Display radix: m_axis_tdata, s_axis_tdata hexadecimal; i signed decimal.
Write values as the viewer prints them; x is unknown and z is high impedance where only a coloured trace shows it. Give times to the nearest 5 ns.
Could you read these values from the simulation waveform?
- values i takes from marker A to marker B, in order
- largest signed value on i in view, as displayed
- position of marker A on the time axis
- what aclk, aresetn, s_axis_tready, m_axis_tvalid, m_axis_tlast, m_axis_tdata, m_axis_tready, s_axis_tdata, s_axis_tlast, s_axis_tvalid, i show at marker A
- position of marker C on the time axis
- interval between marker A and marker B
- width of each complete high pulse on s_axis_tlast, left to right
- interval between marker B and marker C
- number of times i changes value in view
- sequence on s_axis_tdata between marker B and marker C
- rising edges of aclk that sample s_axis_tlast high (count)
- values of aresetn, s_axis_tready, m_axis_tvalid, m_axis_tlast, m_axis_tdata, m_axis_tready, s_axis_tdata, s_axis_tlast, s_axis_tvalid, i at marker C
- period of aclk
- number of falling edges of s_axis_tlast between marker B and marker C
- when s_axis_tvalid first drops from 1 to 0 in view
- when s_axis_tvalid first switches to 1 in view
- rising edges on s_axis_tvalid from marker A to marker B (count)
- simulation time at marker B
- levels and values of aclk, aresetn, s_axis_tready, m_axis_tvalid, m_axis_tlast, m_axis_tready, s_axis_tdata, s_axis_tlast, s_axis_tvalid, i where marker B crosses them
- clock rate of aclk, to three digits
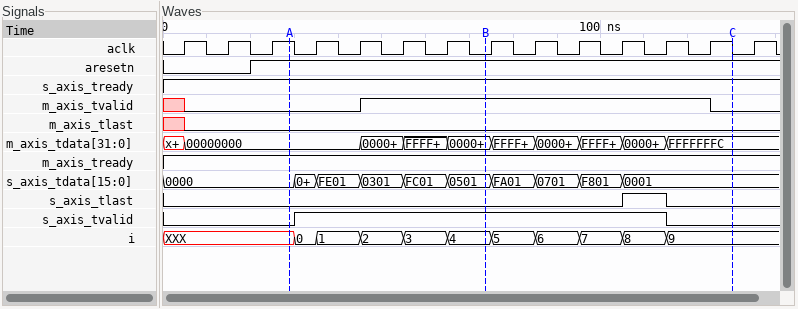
XXX, 0, 1, 2, 3, 4
9
30 ns
aclk=1, aresetn=1, s_axis_tready=1, m_axis_tvalid=0, m_axis_tlast=0, m_axis_tdata=00000000, m_axis_tready=1, s_axis_tdata=0000, s_axis_tlast=0, s_axis_tvalid=0, i=XXX
130 ns
45 ns
10 ns
55 ns
10
0501, FA01, 0701, F801, 0001
1
aresetn=1, s_axis_tready=1, m_axis_tvalid=0, m_axis_tlast=0, m_axis_tdata=FFFFFFFC, m_axis_tready=1, s_axis_tdata=0001, s_axis_tlast=0, s_axis_tvalid=0, i=9
10 ns
1
115 ns
30 ns
1
75 ns
aclk=0, aresetn=1, s_axis_tready=1, m_axis_tvalid=1, m_axis_tlast=0, m_axis_tready=1, s_axis_tdata=0501, s_axis_tlast=0, s_axis_tvalid=1, i=4
100 MHz
